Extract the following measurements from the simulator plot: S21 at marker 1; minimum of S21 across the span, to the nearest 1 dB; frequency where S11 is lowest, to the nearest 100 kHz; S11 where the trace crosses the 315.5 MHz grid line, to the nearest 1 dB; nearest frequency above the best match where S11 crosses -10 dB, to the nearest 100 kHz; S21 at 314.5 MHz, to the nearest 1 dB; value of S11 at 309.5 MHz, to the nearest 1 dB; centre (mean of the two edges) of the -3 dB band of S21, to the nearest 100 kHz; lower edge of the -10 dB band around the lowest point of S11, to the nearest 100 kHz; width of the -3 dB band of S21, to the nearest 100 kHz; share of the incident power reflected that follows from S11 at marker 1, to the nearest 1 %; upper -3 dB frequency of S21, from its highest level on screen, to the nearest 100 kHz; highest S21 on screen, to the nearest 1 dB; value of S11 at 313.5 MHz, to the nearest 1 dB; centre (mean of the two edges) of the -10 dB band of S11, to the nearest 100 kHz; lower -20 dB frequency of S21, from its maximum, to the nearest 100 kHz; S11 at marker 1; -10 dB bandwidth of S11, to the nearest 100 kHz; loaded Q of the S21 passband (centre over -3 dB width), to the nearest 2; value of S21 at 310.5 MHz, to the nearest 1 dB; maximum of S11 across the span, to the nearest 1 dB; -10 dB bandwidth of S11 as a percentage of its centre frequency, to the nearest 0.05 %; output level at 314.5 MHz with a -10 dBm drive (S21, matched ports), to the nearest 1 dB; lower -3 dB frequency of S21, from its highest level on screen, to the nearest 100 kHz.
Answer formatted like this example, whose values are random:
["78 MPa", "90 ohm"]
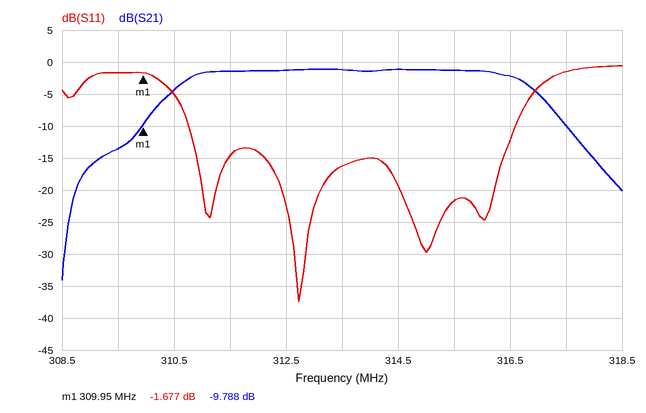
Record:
["-9.788 dB", "-34 dB", "312.7 MHz", "-22 dB", "316.6 MHz", "-1 dB", "-2 dB", "313.7 MHz", "310.8 MHz", "6.4 MHz", "68 %", "316.9 MHz", "-1 dB", "-16 dB", "313.7 MHz", "308.7 MHz", "-1.677 dB", "5.8 MHz", "50", "-4 dB", "-1 dB", "1.85 %", "-11 dBm", "310.5 MHz"]
